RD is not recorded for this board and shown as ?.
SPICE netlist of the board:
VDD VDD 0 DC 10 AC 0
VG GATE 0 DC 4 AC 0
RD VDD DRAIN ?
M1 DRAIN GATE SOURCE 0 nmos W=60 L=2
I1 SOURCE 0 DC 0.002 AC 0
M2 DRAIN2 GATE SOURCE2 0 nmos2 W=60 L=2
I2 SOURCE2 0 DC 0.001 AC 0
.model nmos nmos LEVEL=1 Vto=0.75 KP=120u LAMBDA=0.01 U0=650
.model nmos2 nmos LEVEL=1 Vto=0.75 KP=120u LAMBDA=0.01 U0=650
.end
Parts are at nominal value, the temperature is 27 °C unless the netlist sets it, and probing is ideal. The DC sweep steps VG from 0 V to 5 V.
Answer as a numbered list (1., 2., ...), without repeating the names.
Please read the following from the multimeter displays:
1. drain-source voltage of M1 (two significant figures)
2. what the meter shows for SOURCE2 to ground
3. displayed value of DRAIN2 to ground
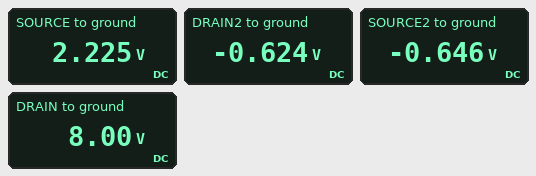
1. 5.8 V
2. -0.646 V
3. -0.624 V
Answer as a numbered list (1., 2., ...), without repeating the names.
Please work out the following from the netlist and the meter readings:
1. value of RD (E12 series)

1. 1 kΩ
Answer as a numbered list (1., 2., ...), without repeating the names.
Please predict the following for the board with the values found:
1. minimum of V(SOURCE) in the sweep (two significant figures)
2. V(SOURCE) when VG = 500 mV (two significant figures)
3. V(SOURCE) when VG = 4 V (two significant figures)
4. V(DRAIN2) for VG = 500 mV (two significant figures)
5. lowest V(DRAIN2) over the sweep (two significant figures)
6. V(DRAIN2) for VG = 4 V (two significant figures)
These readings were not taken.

1. -670 mV
2. -670 mV
3. 2.2 V
4. -590 mV
5. -630 mV
6. -620 mV
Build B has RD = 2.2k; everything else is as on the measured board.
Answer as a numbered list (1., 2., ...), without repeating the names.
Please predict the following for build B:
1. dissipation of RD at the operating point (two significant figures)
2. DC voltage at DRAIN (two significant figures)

1. 8.8 mW
2. 5.6 V
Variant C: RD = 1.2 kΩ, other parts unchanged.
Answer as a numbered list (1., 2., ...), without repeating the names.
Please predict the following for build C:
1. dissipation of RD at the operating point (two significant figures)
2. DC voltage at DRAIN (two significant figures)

1. 4.8 mW
2. 7.6 V
